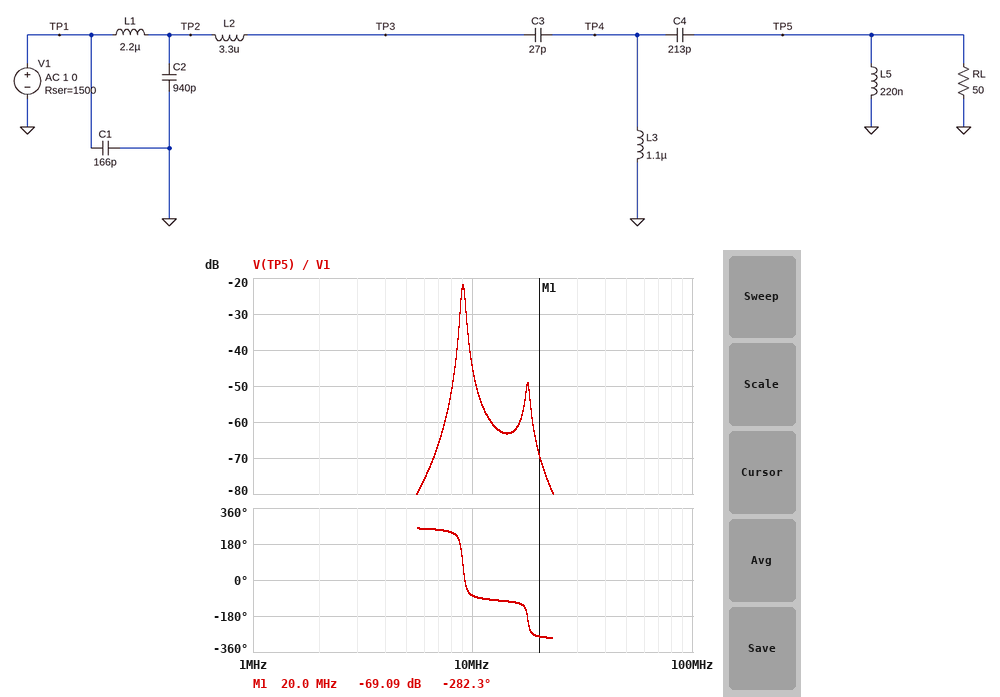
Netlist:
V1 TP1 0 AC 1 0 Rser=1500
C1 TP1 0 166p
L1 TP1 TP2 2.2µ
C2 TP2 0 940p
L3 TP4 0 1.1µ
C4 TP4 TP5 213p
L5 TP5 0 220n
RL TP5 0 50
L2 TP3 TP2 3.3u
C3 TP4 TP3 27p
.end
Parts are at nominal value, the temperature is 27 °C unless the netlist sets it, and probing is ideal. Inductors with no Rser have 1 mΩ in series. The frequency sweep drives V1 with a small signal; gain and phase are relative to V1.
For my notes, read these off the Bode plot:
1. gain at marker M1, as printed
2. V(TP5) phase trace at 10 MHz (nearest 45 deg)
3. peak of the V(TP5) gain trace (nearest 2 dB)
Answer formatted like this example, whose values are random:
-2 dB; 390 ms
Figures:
-69.09 dB; -90 deg; -22 dB
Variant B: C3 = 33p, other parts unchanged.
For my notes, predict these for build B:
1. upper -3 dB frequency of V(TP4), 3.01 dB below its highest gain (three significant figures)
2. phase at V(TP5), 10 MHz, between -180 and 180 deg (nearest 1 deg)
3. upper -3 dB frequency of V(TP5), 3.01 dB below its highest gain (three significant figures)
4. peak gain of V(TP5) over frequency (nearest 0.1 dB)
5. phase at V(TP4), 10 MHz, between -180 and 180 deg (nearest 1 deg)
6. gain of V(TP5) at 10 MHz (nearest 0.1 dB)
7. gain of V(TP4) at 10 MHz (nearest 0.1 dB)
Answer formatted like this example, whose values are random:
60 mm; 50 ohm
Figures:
9.07 MHz; -81 deg; 9.09 MHz; -21.4 dB; 117 deg; -44.8 dB; -31.5 dB
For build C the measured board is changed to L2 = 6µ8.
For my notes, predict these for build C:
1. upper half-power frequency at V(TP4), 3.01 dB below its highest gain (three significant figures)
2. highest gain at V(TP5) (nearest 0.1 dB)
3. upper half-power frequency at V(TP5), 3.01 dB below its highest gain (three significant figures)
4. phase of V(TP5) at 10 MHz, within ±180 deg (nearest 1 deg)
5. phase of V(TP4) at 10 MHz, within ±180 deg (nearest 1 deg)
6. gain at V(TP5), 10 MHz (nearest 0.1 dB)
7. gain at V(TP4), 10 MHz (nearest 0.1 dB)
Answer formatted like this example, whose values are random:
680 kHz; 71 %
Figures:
8.93 MHz; -21.4 dB; 8.99 MHz; -84 deg; 114 deg; -43.6 dB; -30.2 dB
